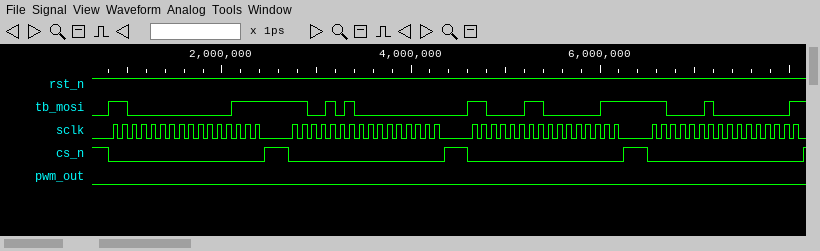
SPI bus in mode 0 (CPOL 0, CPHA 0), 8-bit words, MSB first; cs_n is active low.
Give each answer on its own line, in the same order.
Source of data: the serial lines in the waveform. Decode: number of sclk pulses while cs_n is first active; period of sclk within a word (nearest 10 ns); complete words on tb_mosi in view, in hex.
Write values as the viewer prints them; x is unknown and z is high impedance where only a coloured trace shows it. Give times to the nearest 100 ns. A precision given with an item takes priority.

16
100 ns
C0, 07, CA, 00, C3, 03, C2, 01
